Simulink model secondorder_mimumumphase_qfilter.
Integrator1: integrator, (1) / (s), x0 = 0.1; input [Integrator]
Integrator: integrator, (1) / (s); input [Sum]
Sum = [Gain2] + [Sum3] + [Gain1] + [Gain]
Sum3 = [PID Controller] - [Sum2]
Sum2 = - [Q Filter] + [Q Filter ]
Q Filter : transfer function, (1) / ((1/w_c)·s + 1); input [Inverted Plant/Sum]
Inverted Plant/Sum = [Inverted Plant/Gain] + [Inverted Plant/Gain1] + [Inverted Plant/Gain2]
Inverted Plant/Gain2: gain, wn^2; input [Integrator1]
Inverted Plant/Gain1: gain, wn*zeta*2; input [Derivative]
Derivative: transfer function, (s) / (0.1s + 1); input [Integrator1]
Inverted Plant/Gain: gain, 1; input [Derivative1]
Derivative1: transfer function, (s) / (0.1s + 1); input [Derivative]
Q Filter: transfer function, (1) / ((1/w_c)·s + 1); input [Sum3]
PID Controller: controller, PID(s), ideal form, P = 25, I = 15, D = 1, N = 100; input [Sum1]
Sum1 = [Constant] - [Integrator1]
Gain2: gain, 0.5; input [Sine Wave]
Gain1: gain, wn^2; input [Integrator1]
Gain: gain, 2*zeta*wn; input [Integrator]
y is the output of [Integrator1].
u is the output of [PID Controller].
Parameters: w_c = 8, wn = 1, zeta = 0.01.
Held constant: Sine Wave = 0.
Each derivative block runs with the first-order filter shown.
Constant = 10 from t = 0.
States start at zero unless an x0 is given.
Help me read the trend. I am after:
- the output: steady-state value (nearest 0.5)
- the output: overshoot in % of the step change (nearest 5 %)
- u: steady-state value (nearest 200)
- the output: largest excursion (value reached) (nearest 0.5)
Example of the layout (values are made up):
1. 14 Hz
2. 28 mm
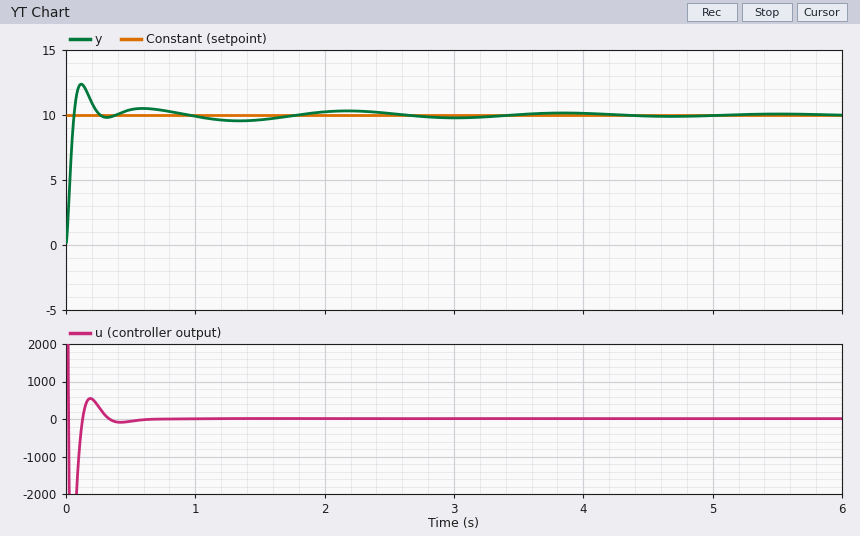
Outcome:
1. 10.0
2. 25 %
3. 0
4. 12.5
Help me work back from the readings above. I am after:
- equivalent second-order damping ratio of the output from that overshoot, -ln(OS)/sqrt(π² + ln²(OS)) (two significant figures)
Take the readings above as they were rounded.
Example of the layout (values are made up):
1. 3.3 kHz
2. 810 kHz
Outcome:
1. 0.40
